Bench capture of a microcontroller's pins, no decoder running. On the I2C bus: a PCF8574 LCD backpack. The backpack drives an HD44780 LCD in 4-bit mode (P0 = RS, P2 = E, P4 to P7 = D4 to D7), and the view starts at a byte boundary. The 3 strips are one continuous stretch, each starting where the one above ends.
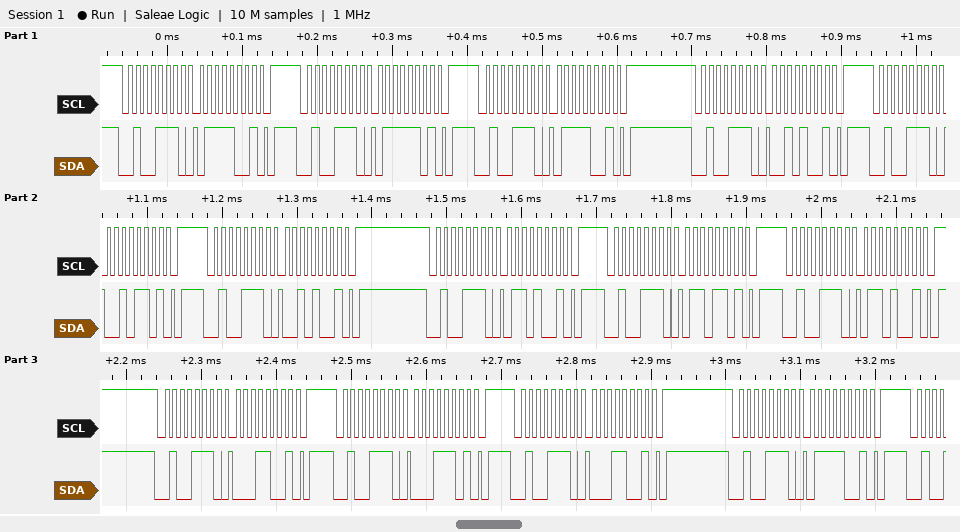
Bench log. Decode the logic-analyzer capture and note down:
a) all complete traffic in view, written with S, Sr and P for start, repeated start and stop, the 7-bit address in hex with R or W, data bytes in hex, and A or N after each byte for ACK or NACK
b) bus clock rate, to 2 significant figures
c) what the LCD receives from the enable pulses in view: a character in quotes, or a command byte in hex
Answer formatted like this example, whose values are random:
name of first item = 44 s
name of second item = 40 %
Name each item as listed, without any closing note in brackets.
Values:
all complete traffic in view, written with S, Sr and P for start, repeated start and stop, the 7-bit address in hex with R or W, data bytes in hex, and A or N after each byte for ACK or NACK = S 27W A 79 A P S 27W A 7D A P S 27W A 79 A P S 27W A 29 A P S 27W A 2D A P S 27W A 29 A P S 27W A 69 A P S 27W A 6D A P S 27W A 69 A P S 27W A 19 A P S 27W A 1D A P S 27W A 19 A P S 27W A 79 A P
bus clock rate, to 2 significant figures = 100 kHz
what the LCD receives from the enable pulses in view: a character in quotes, or a command byte in hex = 'r' 'a'
